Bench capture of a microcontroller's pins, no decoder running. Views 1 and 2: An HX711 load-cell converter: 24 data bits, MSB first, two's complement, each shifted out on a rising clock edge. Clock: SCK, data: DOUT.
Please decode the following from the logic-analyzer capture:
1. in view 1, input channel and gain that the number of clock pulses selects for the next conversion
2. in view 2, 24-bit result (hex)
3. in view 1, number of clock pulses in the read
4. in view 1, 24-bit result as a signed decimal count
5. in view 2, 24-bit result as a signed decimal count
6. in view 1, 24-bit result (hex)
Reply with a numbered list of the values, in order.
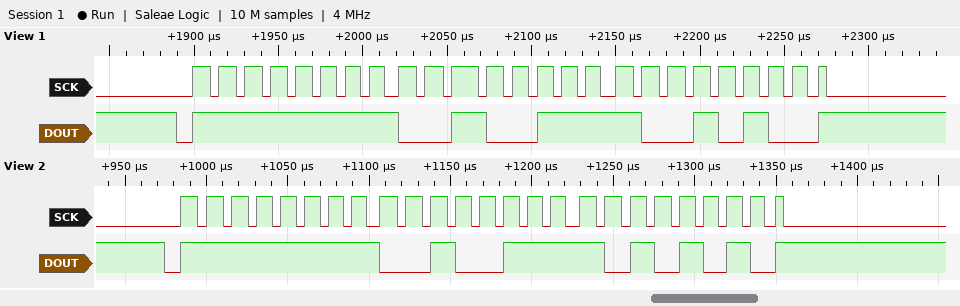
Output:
1. channel A, gain 128
2. 0xFF27AA
3. 25
4. -55404
5. -55382
6. 0xFF2794
